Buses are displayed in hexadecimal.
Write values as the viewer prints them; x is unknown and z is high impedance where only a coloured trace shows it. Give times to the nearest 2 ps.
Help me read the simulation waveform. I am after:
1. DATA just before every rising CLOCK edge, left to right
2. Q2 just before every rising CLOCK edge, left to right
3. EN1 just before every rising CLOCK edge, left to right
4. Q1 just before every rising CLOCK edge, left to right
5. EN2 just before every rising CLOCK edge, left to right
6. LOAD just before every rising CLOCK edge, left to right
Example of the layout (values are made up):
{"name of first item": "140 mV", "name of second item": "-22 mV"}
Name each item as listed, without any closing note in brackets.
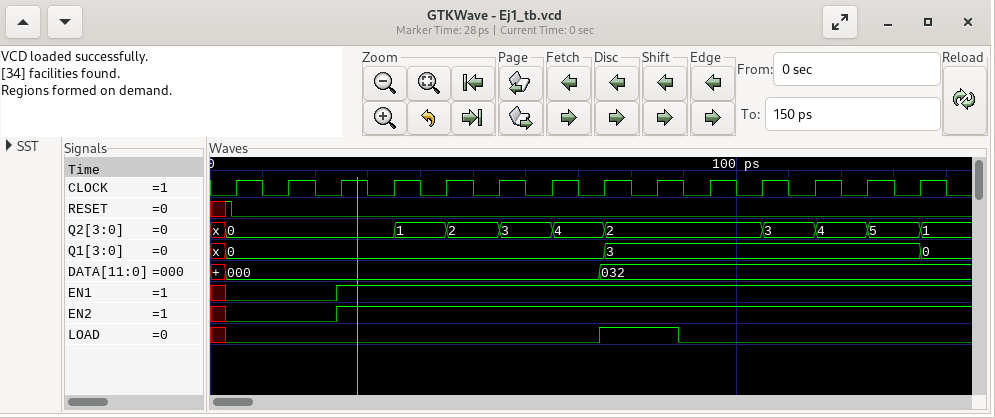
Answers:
{"DATA just before every rising CLOCK edge, left to right": "000, 000, 000, 000, 000, 000, 000, 032, 032, 032, 032, 032, 032, 032", "Q2 just before every rising CLOCK edge, left to right": "0, 0, 0, 0, 1, 2, 3, 4, 2, 2, 2, 3, 4, 5", "EN1 just before every rising CLOCK edge, left to right": "0 0 1 1 1 1 1 1 1 1 1 1 1 1", "Q1 just before every rising CLOCK edge, left to right": "0, 0, 0, 0, 0, 0, 0, 0, 3, 3, 3, 3, 3, 3", "EN2 just before every rising CLOCK edge, left to right": "0 0 1 1 1 1 1 1 1 1 1 1 1 1", "LOAD just before every rising CLOCK edge, left to right": "0 0 0 0 0 0 0 1 1 0 0 0 0 0"}
